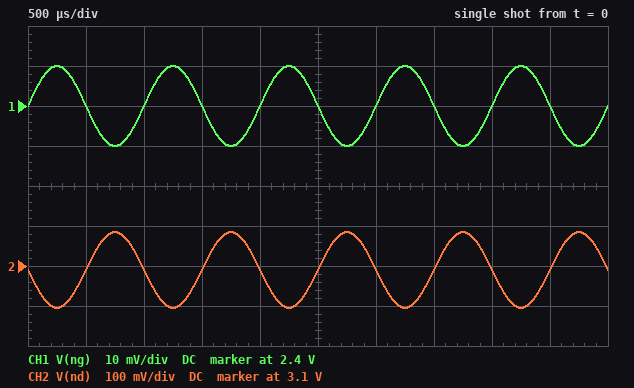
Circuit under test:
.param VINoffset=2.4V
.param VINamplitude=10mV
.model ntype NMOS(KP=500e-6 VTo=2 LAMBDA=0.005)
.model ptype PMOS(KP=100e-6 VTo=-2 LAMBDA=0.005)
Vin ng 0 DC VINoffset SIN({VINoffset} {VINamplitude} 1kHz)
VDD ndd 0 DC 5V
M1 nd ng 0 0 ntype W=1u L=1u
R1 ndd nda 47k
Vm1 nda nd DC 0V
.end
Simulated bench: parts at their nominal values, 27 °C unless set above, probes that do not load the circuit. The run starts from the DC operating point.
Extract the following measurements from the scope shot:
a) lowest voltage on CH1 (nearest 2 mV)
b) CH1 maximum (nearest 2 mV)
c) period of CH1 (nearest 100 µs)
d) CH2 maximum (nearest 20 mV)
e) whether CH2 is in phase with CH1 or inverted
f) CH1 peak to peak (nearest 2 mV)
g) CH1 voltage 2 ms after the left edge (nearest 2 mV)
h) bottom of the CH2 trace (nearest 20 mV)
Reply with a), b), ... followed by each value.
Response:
a) 2.390 V
b) 2.410 V
c) 1.0 ms
d) 3.18 V
e) inverted
f) 20 mV
g) 2.400 V
h) 3.00 V
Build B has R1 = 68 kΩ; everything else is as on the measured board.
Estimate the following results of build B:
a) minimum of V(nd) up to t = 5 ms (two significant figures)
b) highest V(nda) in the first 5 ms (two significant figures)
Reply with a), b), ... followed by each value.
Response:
a) 2.1 V
b) 2.4 V
